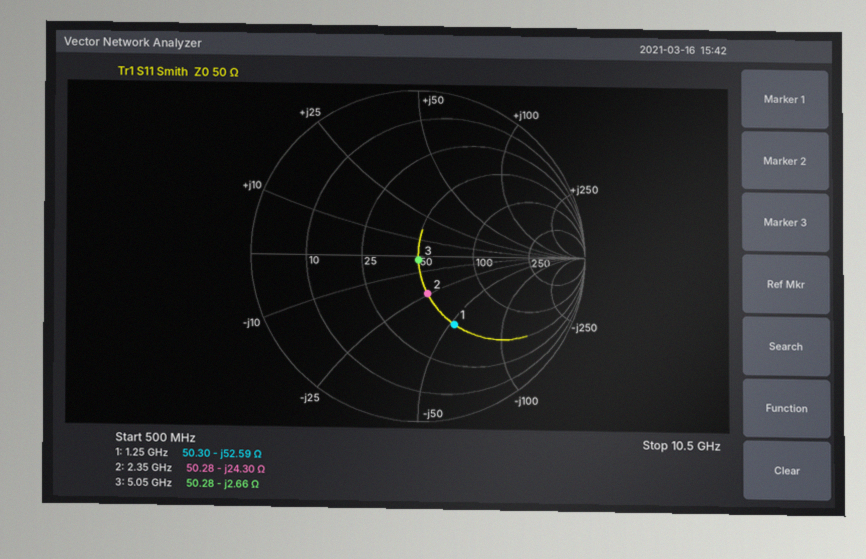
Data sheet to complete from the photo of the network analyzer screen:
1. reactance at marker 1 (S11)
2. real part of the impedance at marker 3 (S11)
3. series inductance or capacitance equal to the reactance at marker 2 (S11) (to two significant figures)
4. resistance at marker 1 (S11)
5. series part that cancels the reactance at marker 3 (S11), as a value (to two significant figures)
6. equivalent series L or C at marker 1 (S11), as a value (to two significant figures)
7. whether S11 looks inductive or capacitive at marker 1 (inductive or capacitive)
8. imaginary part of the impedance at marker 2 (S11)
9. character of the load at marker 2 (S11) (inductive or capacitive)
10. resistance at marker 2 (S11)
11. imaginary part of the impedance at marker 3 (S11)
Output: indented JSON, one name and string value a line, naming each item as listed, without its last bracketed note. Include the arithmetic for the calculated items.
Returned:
{
  "reactance at marker 1": "-52.59 Ω",
  "real part of the impedance at marker 3": "50.28 Ω",
  "series inductance or capacitance equal to the reactance at marker 2 (S11)": "C = 1/(2π × 2.35 GHz × 24.3 Ω) ≈ 2.8 pF",
  "resistance at marker 1": "50.30 Ω",
  "series part that cancels the reactance at marker 3 (S11), as a value": "L = 2.66 Ω/(2π × 5.05 GHz) ≈ 84 pH",
  "equivalent series L or C at marker 1 (S11), as a value": "C = 1/(2π × 1.25 GHz × 52.59 Ω) ≈ 2.4 pF",
  "whether S11 looks inductive or capacitive at marker 1": "capacitive",
  "imaginary part of the impedance at marker 2": "-24.30 Ω",
  "character of the load at marker 2 (S11)": "capacitive",
  "resistance at marker 2": "50.28 Ω",
  "imaginary part of the impedance at marker 3": "-2.66 Ω"
}
